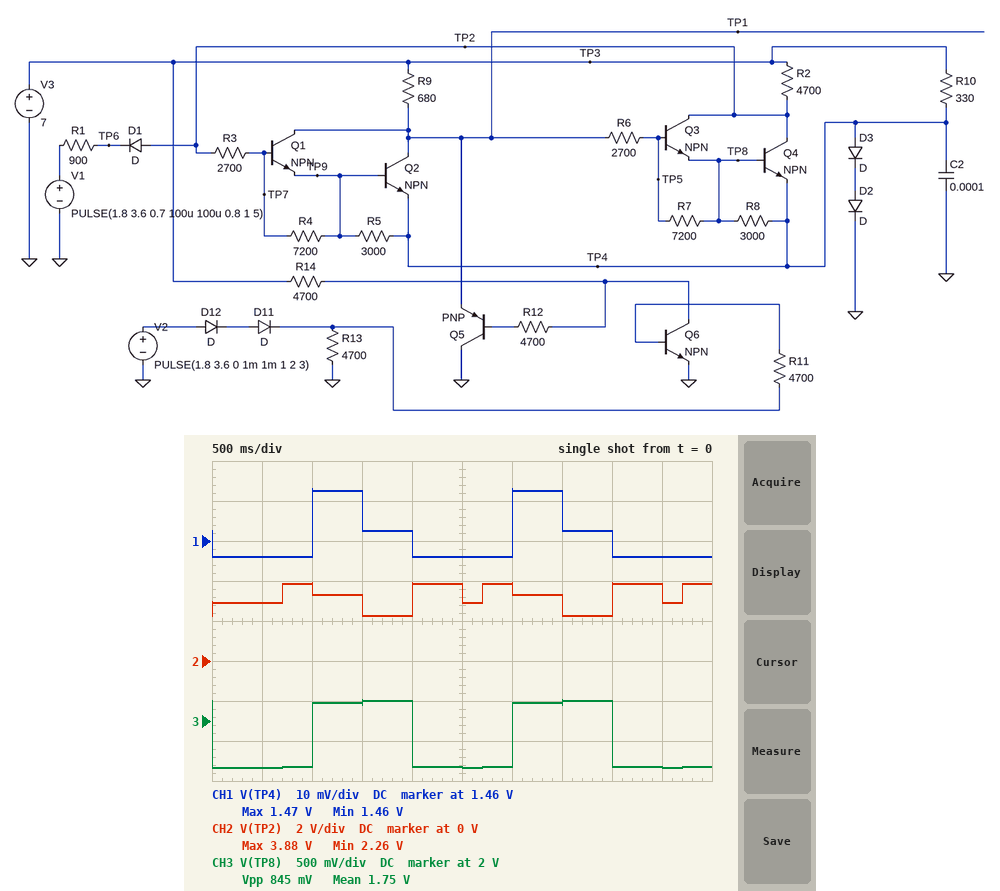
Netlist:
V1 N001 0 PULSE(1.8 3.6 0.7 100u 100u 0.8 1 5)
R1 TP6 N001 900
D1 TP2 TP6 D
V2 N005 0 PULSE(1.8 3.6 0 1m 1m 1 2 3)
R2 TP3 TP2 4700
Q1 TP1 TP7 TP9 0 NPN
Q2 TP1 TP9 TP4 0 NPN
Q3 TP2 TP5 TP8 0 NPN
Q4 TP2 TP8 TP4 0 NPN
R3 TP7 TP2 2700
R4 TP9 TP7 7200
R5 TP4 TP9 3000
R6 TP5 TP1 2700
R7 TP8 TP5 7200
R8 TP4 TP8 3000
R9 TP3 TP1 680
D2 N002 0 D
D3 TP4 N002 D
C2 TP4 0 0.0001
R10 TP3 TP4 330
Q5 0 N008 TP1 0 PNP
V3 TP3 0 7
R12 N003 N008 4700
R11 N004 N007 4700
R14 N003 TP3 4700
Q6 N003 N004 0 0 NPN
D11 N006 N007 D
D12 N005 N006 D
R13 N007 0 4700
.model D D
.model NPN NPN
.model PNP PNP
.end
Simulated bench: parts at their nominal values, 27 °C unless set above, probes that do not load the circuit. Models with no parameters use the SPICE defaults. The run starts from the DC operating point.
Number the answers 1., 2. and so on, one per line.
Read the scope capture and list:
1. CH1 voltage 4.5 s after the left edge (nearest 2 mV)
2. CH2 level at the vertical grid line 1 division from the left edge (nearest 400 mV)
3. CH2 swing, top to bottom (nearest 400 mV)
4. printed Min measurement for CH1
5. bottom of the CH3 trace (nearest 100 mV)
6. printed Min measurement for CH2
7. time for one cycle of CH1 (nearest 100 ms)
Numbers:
1. 1.456 V
2. 2.8 V
3. 1.6 V
4. 1.46 V
5. 1.4 V
6. 2.26 V
7. 2.0 s
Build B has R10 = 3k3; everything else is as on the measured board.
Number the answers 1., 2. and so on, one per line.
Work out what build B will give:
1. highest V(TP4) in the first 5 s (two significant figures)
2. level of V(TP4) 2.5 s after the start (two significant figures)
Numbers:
1. 1.4 V
2. 1.3 V
